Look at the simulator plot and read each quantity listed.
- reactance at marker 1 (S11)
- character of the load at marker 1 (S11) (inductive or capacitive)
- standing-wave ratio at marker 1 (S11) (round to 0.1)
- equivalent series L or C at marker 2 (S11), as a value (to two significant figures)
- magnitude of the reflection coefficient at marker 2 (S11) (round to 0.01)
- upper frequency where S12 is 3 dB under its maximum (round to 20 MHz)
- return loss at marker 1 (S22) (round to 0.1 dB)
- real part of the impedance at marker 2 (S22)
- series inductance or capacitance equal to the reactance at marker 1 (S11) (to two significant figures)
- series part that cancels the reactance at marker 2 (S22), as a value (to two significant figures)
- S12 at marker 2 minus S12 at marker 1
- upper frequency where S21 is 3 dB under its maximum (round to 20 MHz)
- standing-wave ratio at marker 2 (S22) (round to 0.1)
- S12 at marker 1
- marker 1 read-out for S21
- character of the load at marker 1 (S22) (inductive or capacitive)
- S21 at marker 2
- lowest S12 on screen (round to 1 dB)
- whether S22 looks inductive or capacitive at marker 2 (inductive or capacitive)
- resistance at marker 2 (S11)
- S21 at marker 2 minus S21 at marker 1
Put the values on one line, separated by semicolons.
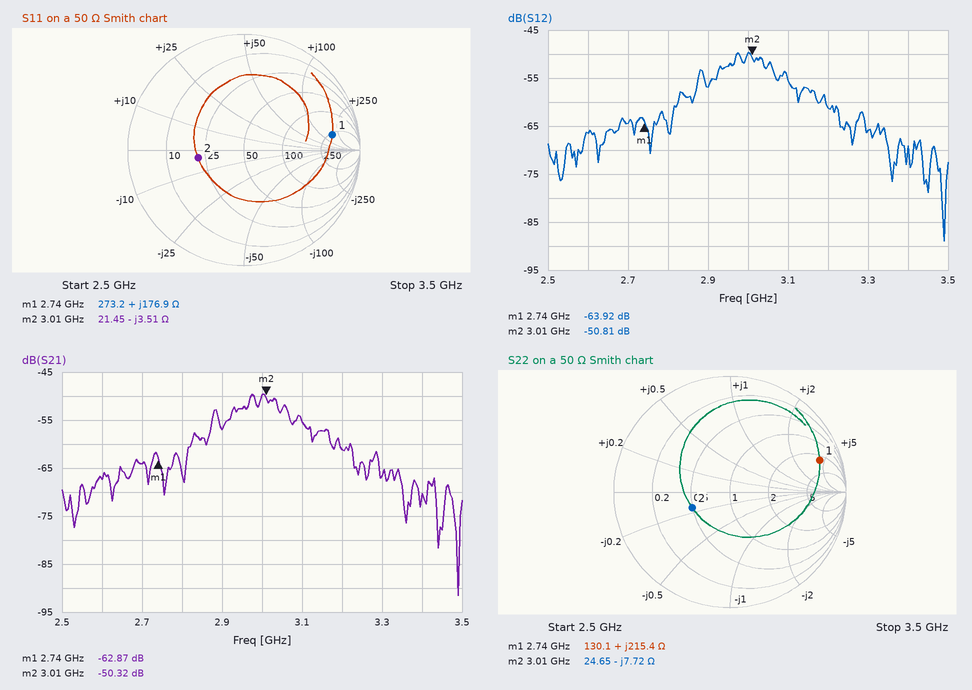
+176.9 Ω; inductive; 7.8; 15 pF; 0.40; 3.04 GHz; 1.7 dB; 24.65 Ω; 10 nH; 410 pH; 13.11 dB; 3.04 GHz; 2.1; -63.92 dB; -62.87 dB; inductive; -50.32 dB; -89 dB; capacitive; 21.45 Ω; 12.55 dB
